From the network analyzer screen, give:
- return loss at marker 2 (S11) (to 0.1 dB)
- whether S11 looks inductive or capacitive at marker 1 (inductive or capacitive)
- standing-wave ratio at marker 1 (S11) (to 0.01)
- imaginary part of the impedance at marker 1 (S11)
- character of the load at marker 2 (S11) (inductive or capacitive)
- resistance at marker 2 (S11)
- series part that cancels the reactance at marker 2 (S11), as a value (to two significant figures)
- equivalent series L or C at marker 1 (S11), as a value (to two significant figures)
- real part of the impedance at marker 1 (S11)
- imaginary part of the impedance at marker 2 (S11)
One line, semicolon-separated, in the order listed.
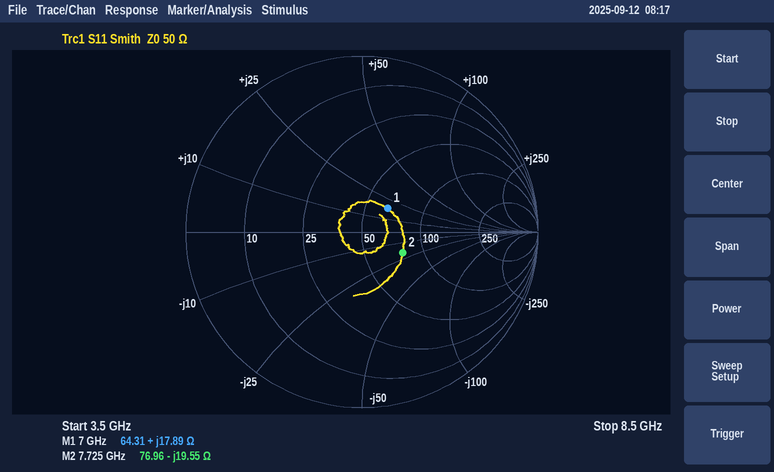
11.7 dB; inductive; 1.49; +17.89 Ω; capacitive; 76.96 Ω; 400 pH; 410 pH; 64.31 Ω; -19.55 Ω
